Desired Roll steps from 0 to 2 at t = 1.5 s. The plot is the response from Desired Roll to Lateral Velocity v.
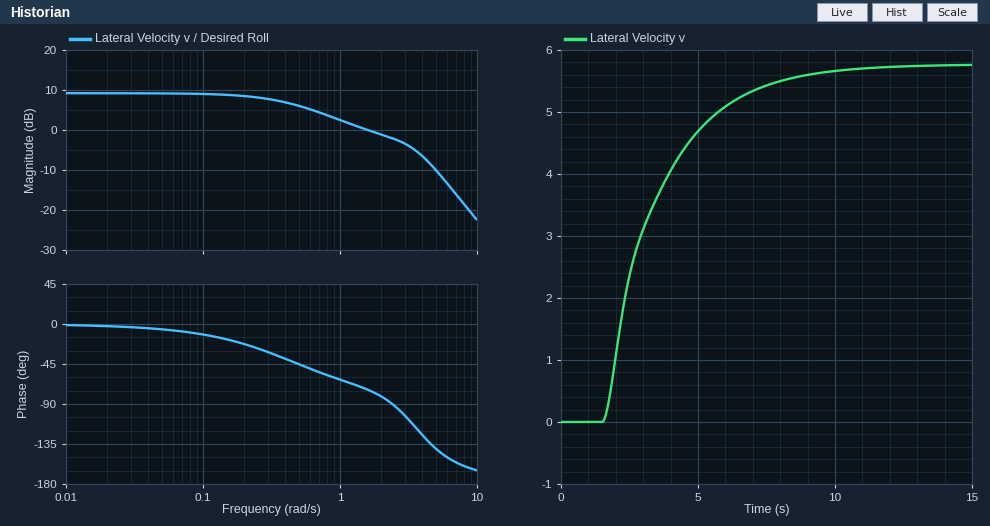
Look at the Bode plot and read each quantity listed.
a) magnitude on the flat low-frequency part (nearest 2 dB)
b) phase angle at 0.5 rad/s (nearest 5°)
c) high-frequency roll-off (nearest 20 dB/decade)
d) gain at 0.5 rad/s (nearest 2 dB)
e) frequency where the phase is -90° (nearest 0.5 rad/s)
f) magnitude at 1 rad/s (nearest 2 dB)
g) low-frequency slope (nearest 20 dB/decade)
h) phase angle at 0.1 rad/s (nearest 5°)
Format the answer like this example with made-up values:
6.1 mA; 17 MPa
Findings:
10 dB; -45°; -40 dB/decade; 6 dB; 2.5 rad/s; 2 dB; 0 dB/decade; -10°
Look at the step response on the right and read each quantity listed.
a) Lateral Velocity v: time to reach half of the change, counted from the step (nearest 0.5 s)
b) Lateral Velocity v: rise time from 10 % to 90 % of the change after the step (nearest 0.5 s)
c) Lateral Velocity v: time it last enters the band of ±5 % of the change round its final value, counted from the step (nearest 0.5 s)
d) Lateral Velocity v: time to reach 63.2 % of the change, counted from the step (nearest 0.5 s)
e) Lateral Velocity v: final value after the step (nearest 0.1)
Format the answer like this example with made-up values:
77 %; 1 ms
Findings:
1.5 s; 4.5 s; 6.5 s; 2.0 s; 5.8
